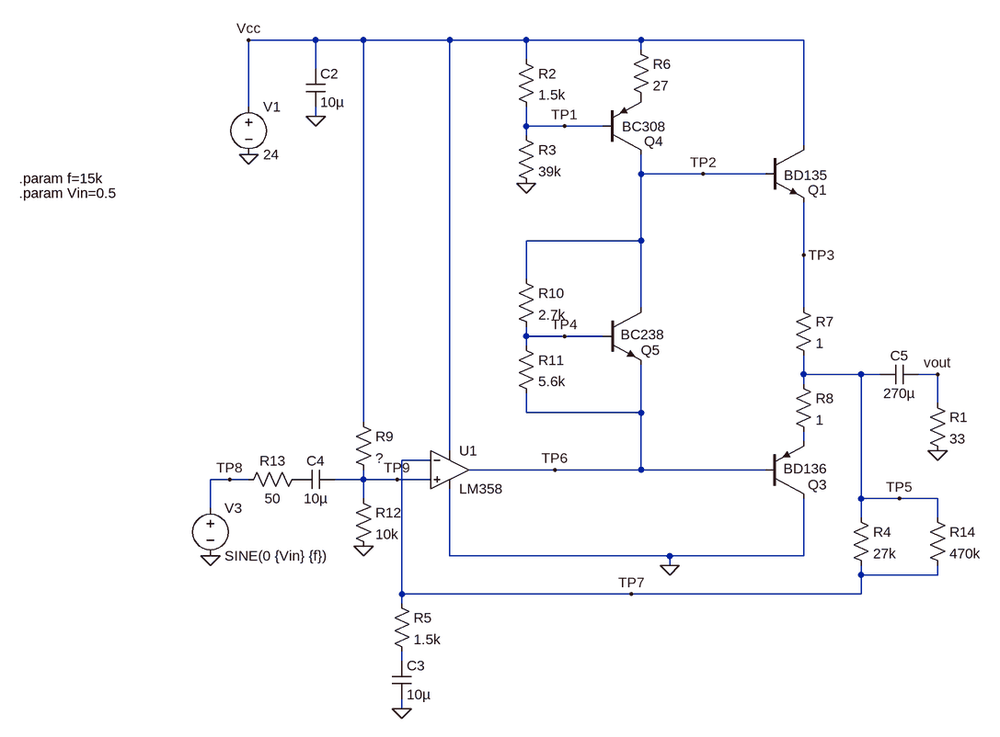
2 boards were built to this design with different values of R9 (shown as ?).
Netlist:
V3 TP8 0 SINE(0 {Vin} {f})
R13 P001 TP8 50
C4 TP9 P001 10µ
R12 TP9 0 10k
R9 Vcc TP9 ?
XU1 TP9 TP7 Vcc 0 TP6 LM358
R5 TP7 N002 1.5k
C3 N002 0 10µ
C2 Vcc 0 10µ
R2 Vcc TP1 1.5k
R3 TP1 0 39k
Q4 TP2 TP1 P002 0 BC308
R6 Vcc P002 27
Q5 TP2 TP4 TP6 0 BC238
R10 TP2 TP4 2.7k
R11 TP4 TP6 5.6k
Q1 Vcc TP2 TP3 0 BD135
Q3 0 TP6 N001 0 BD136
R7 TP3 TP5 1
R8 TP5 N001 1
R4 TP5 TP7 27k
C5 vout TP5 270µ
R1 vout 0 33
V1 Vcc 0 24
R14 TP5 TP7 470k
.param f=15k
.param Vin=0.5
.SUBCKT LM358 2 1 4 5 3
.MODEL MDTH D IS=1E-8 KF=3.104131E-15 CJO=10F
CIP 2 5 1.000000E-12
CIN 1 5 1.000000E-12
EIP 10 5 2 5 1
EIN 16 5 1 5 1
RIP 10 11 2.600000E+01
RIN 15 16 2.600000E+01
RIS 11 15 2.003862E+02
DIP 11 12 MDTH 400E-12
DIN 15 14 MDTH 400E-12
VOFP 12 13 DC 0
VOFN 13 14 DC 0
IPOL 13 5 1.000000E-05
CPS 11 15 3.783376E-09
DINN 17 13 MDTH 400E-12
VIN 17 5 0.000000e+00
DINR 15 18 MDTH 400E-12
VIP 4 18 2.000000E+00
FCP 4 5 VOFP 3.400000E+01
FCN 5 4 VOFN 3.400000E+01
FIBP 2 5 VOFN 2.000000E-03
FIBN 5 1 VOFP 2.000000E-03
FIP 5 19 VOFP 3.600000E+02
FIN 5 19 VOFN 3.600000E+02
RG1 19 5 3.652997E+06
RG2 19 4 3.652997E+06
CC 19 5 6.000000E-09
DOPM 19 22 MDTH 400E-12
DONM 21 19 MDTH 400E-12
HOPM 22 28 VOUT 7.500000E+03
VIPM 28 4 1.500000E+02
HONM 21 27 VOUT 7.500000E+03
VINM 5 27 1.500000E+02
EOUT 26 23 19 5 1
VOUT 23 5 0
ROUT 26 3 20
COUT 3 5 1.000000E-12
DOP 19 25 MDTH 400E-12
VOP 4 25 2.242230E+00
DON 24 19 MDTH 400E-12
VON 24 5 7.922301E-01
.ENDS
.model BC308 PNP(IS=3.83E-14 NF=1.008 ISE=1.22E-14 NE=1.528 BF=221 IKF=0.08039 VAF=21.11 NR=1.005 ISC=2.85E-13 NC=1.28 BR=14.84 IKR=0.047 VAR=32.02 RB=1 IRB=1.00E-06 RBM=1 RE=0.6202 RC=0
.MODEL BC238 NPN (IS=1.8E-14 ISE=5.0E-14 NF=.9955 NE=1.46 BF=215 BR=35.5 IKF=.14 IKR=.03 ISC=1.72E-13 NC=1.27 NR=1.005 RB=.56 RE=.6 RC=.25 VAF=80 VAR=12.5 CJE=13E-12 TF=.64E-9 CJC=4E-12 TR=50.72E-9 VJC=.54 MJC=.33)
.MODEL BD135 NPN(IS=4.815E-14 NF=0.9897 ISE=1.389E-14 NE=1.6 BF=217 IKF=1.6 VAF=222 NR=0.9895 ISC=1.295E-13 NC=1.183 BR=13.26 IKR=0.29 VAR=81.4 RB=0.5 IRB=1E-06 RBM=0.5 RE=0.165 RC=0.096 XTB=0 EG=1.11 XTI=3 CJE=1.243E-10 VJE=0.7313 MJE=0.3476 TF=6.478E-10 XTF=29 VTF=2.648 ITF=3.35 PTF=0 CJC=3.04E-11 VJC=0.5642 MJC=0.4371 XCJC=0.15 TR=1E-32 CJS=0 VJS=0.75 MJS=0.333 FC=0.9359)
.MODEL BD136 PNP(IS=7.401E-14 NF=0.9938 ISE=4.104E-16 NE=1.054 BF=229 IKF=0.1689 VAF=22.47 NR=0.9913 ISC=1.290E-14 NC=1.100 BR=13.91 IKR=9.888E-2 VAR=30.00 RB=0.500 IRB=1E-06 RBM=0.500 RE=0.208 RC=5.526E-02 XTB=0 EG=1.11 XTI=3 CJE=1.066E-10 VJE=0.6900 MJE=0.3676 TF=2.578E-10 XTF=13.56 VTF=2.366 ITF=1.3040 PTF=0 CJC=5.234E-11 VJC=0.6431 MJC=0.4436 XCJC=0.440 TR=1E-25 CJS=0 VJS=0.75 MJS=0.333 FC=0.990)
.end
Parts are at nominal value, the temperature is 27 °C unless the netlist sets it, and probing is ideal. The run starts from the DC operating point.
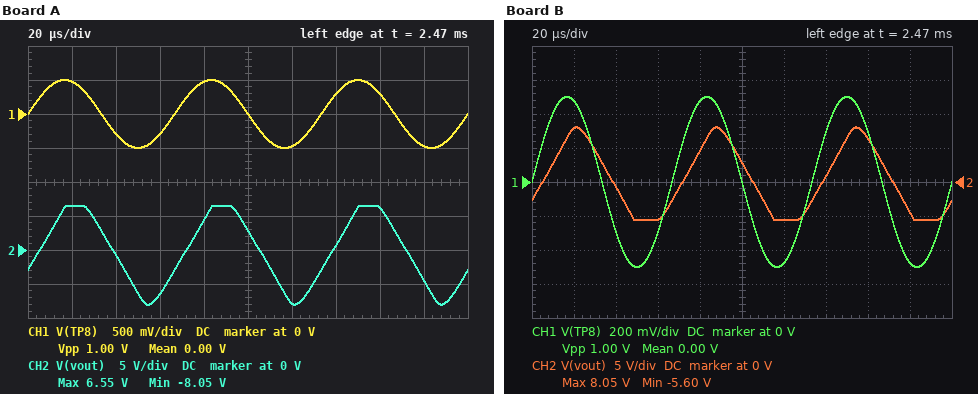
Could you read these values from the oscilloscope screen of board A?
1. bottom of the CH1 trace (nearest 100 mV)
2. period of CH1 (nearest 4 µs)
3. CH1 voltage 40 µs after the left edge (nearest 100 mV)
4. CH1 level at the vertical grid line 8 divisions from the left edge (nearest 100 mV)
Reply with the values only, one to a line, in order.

-500 mV
68 µs
-300 mV
300 mV
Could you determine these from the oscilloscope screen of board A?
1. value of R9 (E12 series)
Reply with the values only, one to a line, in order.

4.7 kΩ
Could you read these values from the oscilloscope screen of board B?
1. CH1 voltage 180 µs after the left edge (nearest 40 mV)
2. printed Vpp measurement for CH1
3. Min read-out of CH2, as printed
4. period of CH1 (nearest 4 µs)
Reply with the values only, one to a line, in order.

-480 mV
1.00 V
-5.60 V
68 µs
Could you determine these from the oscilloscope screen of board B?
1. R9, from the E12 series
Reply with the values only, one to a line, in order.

27 kΩ
